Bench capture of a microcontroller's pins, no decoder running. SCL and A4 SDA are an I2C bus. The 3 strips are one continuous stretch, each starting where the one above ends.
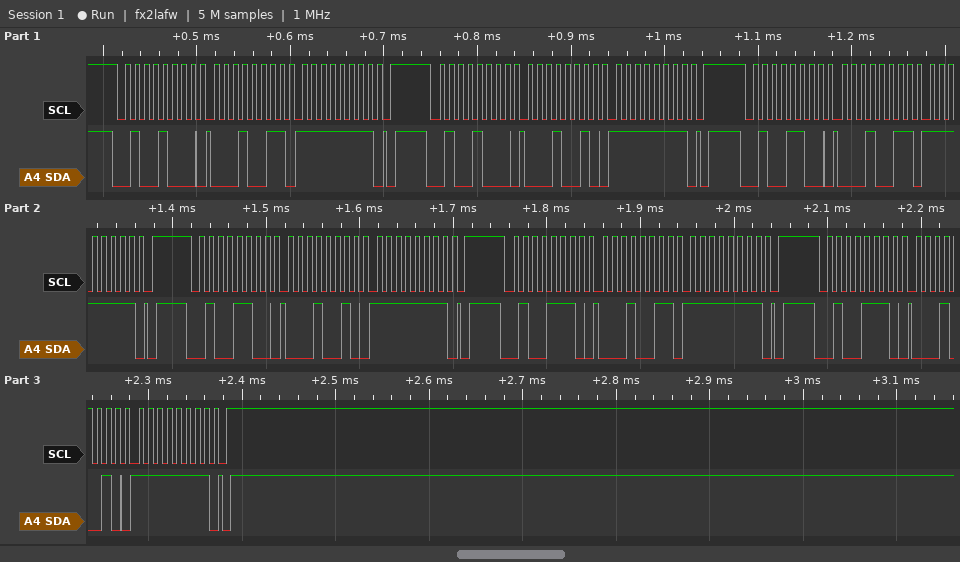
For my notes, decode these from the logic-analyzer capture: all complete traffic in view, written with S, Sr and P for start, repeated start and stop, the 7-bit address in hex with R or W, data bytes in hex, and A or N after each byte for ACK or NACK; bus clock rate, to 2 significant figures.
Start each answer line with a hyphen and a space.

- S 24W A 13 A FF A P S 24W A 12 A FF A P S 26W A 13 A FF A P S 26W A 12 A FF A P S 27W A 13 A FF A P S 27W A 12 A FF A P
- 100 kHz
